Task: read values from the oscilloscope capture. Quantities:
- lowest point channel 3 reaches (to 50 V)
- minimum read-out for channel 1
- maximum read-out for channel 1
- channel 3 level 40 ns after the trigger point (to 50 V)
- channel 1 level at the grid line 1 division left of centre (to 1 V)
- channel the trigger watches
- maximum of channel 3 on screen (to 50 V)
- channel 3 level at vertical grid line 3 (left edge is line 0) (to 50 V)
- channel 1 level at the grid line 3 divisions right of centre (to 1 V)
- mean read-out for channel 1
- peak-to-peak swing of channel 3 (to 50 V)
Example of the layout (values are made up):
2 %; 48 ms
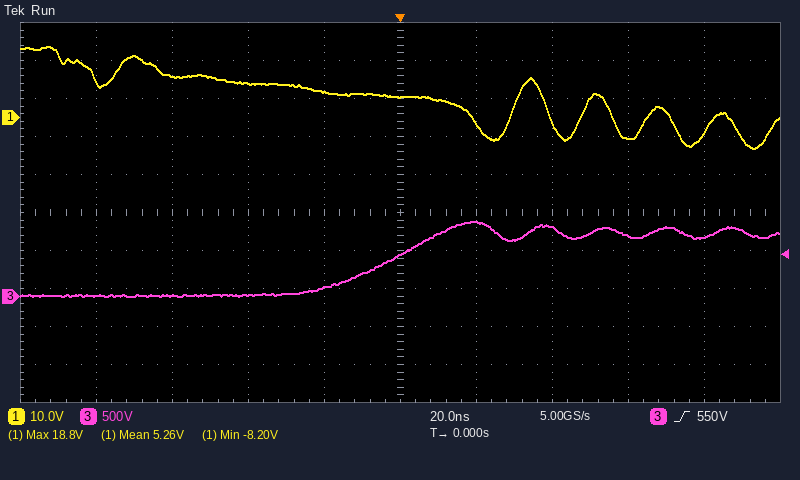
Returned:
0 V; -8.20 V; 18.8 V; 900 V; 7 V; channel 3; 1.00 kV; 0 V; -5 V; 5.26 V; 1.00 kV
